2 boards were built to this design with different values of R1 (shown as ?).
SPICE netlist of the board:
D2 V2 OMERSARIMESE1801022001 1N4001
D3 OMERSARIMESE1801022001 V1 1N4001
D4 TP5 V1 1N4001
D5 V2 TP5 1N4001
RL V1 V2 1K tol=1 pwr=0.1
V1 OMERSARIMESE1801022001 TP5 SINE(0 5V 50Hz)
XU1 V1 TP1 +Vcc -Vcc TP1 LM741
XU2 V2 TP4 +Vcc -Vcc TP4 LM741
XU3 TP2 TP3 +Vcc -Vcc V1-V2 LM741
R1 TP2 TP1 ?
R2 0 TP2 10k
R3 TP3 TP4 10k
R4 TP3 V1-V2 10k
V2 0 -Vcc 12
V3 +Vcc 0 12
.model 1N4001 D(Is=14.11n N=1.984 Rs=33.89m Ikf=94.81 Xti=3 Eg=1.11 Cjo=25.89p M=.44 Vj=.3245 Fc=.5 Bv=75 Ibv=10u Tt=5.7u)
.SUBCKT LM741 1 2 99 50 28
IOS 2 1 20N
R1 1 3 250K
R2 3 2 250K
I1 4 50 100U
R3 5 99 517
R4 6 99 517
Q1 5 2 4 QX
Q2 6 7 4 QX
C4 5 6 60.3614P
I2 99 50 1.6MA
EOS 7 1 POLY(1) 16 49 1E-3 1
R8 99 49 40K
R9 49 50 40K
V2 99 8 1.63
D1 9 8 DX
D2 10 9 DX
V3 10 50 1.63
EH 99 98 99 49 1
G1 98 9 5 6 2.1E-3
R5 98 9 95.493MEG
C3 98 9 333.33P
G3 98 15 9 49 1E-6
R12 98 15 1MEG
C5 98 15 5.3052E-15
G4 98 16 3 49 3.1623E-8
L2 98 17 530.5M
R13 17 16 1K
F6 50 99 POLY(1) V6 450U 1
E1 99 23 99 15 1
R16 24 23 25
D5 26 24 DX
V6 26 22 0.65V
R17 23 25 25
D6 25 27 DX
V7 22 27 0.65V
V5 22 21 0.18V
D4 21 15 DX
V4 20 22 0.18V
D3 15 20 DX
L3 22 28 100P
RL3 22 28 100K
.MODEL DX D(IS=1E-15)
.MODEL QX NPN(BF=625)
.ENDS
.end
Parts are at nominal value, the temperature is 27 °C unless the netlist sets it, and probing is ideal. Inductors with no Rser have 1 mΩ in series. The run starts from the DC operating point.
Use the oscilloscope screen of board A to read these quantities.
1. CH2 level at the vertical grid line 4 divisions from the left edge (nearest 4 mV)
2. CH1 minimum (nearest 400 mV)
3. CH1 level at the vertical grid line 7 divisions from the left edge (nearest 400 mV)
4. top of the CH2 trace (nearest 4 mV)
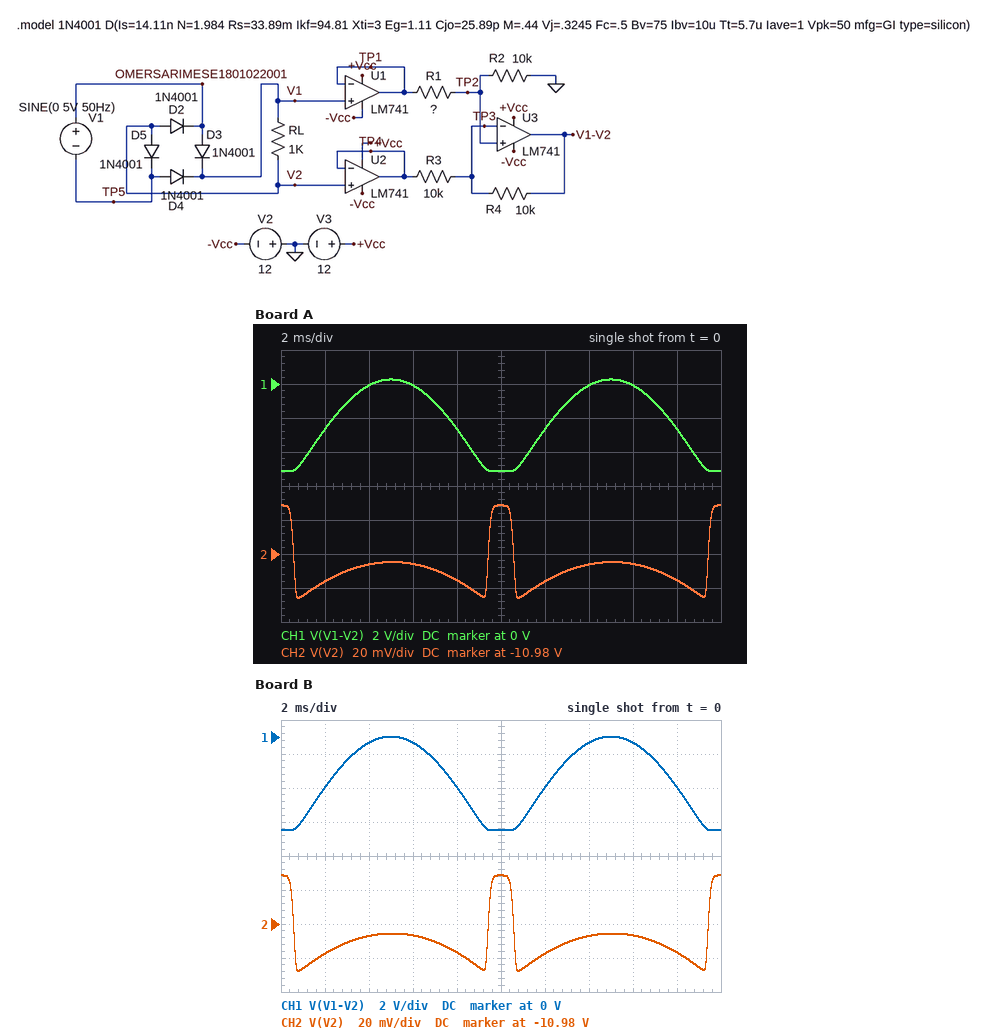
-10.996 V
-5.2 V
0 V
-10.952 V
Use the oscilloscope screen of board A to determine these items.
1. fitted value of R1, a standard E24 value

3.6 kΩ
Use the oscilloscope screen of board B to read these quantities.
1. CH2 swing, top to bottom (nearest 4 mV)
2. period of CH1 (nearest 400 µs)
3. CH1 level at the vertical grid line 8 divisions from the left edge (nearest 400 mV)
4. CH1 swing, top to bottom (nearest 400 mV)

56 mV
10.0 ms
-400 mV
5.6 V
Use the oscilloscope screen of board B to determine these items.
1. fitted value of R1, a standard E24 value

3.3 kΩ
